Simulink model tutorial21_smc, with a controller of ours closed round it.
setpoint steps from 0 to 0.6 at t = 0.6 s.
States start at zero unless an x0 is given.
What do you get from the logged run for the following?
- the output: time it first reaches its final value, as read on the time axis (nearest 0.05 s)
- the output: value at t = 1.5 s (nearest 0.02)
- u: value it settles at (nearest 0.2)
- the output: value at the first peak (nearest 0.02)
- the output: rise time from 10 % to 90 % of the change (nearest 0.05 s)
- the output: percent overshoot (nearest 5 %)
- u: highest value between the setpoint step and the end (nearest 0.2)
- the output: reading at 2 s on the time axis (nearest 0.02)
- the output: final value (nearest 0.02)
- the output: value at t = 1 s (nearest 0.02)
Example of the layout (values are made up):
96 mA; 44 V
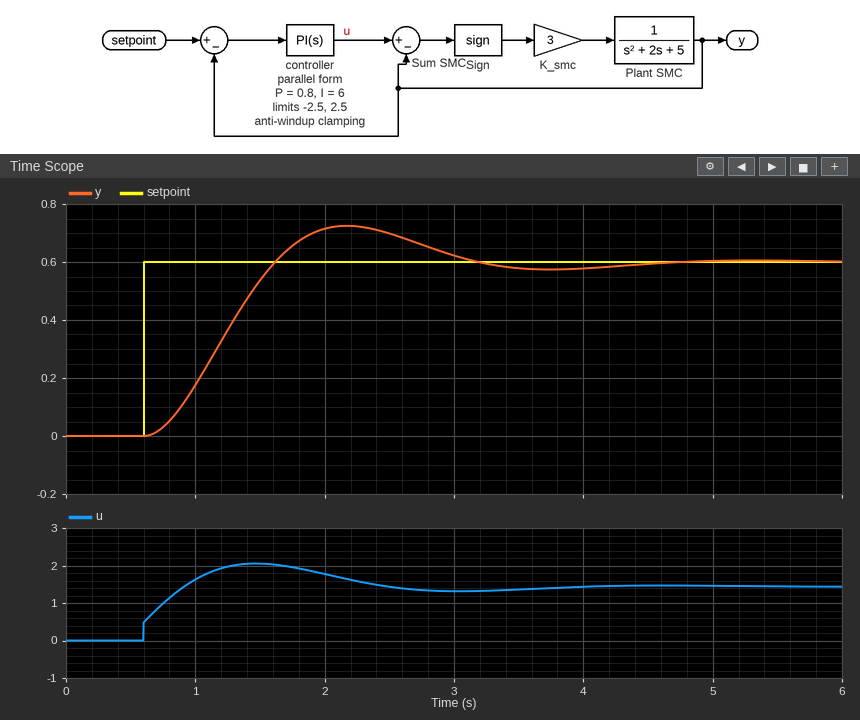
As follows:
1.60 s; 0.54; 1.4; 0.72; 0.70 s; 20 %; 2.0; 0.72; 0.60; 0.18
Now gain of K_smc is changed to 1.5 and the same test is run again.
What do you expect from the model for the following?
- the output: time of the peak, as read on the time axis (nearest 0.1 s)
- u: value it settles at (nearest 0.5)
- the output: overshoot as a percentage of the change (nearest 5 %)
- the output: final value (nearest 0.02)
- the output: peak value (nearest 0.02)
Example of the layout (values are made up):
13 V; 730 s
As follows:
2.2 s; 2.5; 20 %; 0.30; 0.36
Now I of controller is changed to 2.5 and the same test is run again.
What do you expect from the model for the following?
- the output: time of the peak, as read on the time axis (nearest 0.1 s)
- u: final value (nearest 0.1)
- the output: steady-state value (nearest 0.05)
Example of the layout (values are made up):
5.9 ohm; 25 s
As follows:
2.0 s; 0.9; 0.60
